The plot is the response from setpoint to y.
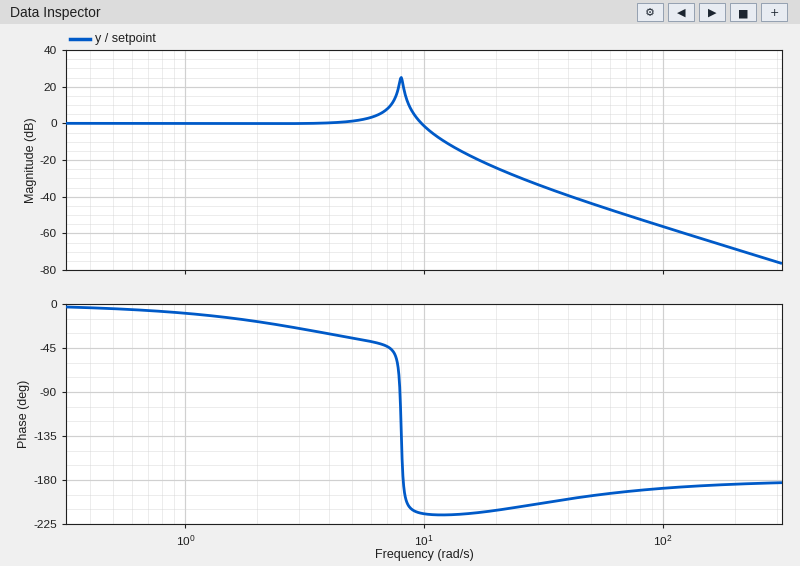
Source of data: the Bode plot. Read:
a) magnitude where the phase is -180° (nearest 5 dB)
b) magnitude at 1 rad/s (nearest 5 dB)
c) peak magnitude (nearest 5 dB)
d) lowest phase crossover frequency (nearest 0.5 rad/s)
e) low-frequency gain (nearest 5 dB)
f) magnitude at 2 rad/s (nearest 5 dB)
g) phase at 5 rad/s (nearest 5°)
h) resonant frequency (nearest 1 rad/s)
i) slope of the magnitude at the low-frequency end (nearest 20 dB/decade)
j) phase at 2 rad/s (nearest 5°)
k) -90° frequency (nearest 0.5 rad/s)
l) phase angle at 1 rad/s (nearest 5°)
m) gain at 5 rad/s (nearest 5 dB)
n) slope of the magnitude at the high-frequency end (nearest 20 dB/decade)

20 dB
0 dB
25 dB
8.0 rad/s
0 dB
0 dB
-35°
8 rad/s
0 dB/decade
-20°
8.0 rad/s
-10°
0 dB
-40 dB/decade
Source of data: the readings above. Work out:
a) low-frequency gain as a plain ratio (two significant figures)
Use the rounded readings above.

1.0
